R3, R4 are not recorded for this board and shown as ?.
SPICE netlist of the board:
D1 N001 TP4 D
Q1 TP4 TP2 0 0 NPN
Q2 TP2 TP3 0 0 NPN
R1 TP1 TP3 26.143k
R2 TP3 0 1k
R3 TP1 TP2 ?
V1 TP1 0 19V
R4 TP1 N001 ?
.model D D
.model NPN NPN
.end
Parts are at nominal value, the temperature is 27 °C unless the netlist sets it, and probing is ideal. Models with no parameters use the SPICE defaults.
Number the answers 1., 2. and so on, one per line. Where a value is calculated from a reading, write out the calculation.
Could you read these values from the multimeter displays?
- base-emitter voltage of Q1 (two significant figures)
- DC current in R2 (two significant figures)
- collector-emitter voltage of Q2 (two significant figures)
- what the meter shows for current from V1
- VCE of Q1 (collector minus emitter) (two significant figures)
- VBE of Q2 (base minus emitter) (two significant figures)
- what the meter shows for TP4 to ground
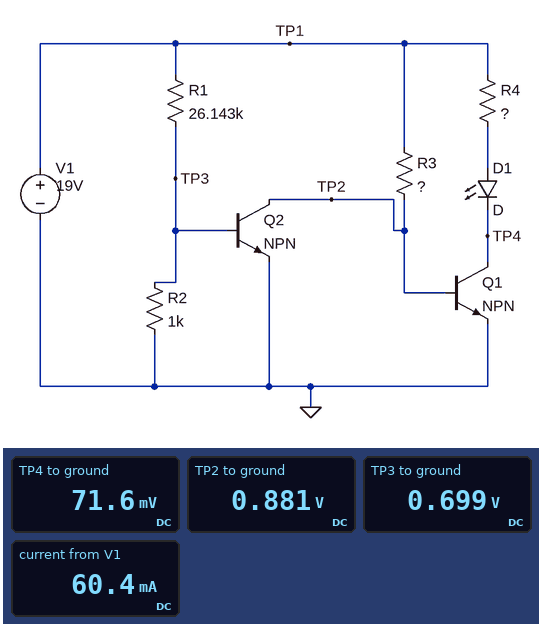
1. 881 mV = 880 mV
2. (699 mV) / 1 kΩ = 700 µA
3. 881 mV = 880 mV
4. 60.4 mA
5. 71.6 mV = 72 mV
6. 699 mV = 700 mV
7. 71.6 mV
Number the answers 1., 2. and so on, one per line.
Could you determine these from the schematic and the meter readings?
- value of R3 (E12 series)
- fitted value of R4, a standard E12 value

1. 3.9 kΩ
2. 330 Ω
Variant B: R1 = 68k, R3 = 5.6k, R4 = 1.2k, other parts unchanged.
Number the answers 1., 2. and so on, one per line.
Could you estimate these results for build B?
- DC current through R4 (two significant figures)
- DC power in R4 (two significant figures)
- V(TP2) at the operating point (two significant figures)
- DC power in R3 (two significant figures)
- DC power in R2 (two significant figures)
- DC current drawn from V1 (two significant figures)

1. 15 mA
2. 280 mW
3. 850 mV
4. 59 mW
5. 76 µW
6. 19 mA
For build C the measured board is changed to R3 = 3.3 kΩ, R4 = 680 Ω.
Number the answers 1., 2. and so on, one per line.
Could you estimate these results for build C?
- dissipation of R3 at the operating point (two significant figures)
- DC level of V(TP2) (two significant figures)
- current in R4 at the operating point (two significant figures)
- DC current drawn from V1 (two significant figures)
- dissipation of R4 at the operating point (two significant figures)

1. 100 mW
2. 870 mV
3. 27 mA
4. 33 mA
5. 490 mW
